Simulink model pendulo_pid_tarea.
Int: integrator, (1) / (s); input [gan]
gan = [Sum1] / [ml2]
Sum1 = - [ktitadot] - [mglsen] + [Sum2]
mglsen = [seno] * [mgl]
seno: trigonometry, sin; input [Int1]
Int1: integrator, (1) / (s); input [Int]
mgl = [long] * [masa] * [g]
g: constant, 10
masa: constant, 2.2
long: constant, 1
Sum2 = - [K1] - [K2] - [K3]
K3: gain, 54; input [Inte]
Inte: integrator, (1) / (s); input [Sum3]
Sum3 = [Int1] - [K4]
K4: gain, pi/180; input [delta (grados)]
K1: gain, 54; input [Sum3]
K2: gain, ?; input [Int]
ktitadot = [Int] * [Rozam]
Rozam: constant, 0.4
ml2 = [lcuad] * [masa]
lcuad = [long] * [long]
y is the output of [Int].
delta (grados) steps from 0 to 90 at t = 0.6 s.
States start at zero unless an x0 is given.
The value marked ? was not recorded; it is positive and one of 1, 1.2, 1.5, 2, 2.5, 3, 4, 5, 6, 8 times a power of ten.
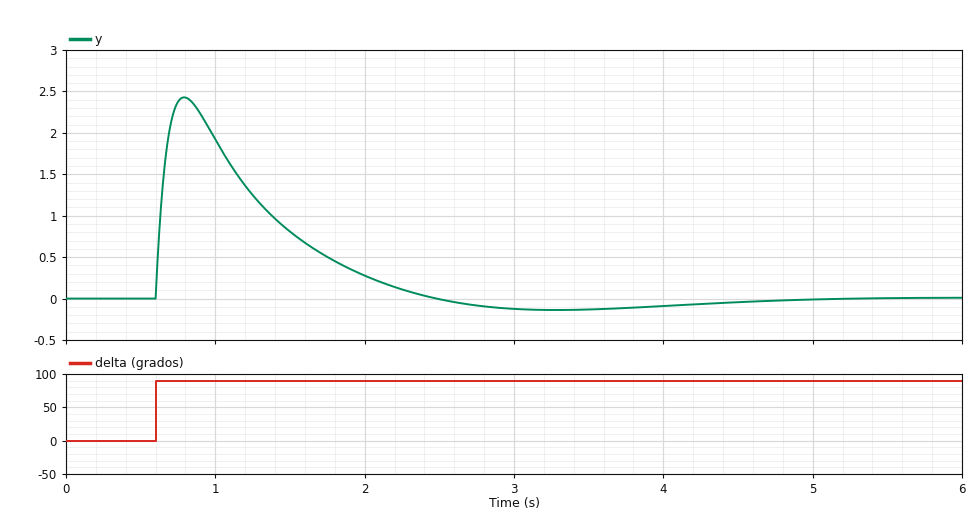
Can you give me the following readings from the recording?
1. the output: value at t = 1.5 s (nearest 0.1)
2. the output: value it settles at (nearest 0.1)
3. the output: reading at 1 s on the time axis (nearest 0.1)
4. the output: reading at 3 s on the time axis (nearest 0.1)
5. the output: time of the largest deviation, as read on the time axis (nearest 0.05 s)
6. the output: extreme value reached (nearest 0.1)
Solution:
0.8
0.0
1.9
-0.1
0.80 s
2.4
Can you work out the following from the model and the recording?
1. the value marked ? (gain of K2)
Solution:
30
